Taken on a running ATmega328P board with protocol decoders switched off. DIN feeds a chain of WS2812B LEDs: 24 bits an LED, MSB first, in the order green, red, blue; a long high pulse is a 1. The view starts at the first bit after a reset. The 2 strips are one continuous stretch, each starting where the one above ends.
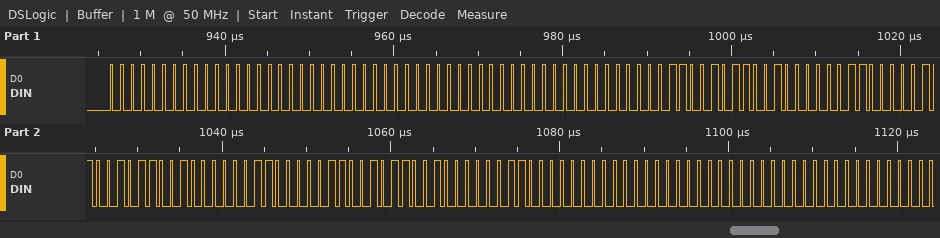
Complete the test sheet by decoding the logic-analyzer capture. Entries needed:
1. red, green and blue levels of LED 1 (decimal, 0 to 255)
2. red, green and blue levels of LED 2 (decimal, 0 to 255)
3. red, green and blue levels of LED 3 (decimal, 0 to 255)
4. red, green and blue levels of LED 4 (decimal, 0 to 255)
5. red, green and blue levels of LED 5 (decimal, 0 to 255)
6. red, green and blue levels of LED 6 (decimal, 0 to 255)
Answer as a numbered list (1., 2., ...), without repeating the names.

1. 0, 0, 0
2. 0, 0, 0
3. 89, 6, 3
4. 89, 6, 3
5. 89, 6, 3
6. 0, 0, 0
